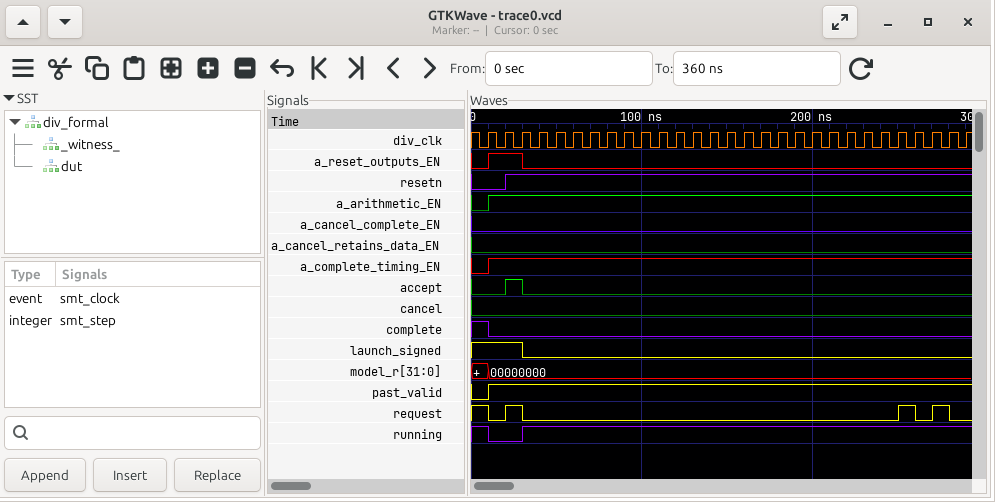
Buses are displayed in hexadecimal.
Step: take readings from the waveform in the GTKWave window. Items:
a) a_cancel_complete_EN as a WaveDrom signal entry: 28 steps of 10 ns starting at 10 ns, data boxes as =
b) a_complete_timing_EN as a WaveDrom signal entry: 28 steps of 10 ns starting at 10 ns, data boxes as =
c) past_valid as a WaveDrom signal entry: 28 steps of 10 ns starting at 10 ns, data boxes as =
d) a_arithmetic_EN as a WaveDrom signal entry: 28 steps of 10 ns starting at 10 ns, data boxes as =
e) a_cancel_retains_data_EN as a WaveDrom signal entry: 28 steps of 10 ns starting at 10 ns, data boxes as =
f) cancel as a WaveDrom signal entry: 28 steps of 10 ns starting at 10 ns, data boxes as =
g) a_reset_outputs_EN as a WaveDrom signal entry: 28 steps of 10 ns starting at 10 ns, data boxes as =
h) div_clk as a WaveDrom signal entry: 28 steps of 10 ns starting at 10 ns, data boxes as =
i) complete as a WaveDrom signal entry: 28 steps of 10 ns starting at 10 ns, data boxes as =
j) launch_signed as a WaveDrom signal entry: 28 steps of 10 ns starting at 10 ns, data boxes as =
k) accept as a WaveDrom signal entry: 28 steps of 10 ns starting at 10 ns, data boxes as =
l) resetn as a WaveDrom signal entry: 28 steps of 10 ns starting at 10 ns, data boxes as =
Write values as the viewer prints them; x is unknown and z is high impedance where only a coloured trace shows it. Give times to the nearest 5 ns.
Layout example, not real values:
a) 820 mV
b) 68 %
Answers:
a) {name: 'a_cancel_complete_EN', wave: '0...........................'}
b) {name: 'a_complete_timing_EN', wave: '1...........................'}
c) {name: 'past_valid', wave: '1...........................'}
d) {name: 'a_arithmetic_EN', wave: '1...........................'}
e) {name: 'a_cancel_retains_data_EN', wave: '0...........................'}
f) {name: 'cancel', wave: '0...........................'}
g) {name: 'a_reset_outputs_EN', wave: '1.0.........................'}
h) {name: 'div_clk', wave: 'p...........................'}
i) {name: 'complete', wave: '0...........................'}
j) {name: 'launch_signed', wave: '1.0.........................'}
k) {name: 'accept', wave: '010.........................'}
l) {name: 'resetn', wave: '01..........................'}
